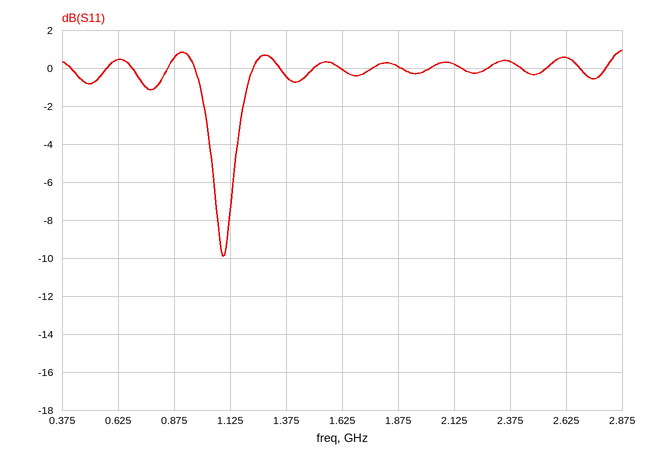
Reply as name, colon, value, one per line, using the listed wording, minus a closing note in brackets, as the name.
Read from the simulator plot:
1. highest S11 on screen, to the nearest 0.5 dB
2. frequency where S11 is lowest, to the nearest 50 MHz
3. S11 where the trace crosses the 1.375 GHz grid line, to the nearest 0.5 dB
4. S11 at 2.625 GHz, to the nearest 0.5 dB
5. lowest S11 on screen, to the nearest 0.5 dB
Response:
highest S11 on screen, to the nearest 0.5 dB: 1.0 dB
frequency where S11 is lowest, to the nearest 50 MHz: 1.10 GHz
S11 where the trace crosses the 1.375 GHz grid line, to the nearest 0.5 dB: -0.5 dB
S11 at 2.625 GHz, to the nearest 0.5 dB: 0.5 dB
lowest S11 on screen, to the nearest 0.5 dB: -10.0 dB
